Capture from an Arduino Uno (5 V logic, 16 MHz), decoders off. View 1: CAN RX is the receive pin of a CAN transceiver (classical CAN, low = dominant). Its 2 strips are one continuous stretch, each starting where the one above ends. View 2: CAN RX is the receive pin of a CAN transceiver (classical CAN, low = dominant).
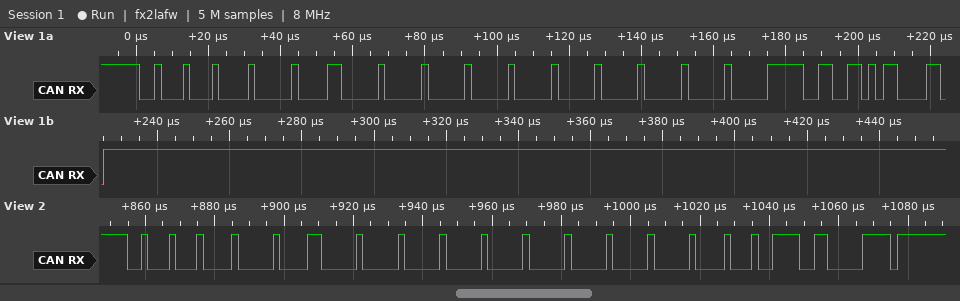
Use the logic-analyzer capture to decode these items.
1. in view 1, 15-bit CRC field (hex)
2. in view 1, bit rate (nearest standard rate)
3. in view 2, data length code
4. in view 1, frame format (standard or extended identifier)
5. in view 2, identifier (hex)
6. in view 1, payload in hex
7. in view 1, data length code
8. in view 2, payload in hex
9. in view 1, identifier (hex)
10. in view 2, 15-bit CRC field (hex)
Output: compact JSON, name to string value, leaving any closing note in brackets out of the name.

{"in view 1, 15-bit CRC field": "0x4D61", "in view 1, bit rate": "500 kbit/s", "in view 2, data length code": "8", "in view 1, frame format": "standard", "in view 2, identifier": "0x222", "in view 1, payload in hex": "03 00 00 00 00 00 00 3D", "in view 1, data length code": "8", "in view 2, payload in hex": "03 00 00 00 00 00 00 44", "in view 1, identifier": "0x222", "in view 2, 15-bit CRC field": "0x7983"}
